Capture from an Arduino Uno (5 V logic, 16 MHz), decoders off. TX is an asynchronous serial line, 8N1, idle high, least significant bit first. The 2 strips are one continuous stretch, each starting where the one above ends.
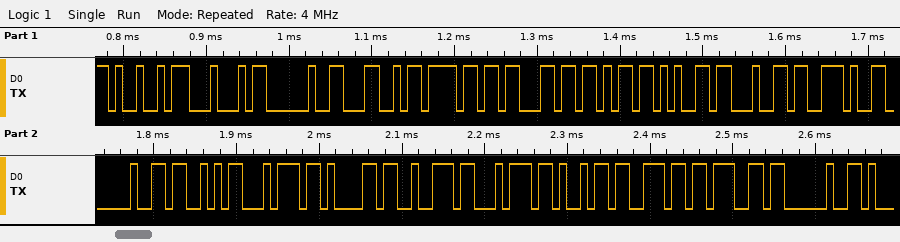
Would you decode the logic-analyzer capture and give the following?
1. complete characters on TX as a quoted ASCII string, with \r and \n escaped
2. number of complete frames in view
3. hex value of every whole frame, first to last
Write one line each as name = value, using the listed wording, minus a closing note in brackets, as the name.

complete characters on TX as a quoted ASCII string, with \r and \n escaped = "ID Locked. Starting "
number of complete frames in view = 20
hex value of every whole frame, first to last = 49 44 20 4C 6F 63 6B 65 64 2E 20 53 74 61 72 74 69 6E 67 20
